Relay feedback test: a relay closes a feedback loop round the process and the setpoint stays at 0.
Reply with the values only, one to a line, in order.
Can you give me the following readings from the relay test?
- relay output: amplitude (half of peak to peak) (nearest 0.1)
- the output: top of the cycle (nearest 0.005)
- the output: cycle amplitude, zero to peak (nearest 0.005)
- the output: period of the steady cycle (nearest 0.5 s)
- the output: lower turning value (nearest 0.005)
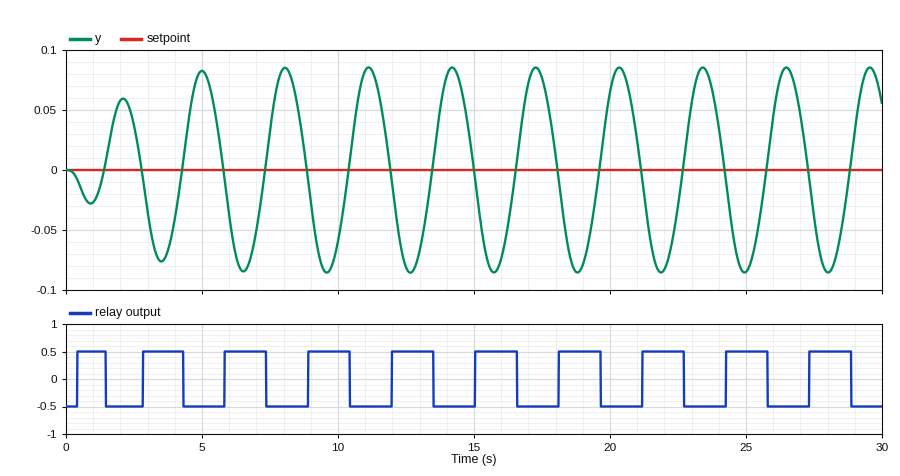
0.5
0.085
0.085
3.0 s
-0.085
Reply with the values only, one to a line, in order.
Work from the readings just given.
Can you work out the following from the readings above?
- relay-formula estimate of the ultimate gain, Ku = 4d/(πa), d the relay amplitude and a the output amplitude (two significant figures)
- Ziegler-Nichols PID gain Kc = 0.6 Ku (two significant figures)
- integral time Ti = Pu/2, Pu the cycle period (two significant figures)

7.5
4.5
1.5 s
